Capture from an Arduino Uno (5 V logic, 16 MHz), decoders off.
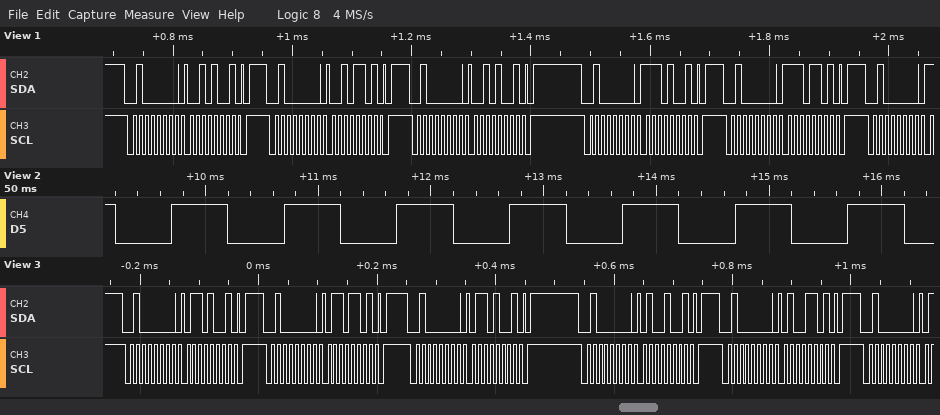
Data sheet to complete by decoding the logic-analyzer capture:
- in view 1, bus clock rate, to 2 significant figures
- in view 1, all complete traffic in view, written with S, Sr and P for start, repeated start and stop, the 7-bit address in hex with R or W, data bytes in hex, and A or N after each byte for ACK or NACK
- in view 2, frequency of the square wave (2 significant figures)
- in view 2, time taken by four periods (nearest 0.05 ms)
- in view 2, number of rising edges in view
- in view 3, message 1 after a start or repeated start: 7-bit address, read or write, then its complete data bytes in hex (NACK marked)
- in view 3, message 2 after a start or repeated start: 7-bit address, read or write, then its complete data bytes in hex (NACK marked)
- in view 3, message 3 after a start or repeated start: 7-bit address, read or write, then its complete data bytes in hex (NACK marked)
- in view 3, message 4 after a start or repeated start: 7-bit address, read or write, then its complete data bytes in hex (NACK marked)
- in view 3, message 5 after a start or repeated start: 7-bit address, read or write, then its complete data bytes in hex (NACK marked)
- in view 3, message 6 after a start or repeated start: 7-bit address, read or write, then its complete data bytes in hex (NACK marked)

100 kHz
S 20W A 29 A P S 20W A 2D A P S 20W A 29 A P S 20W A E9 A P S 20W A ED A P S 20W A
1.0 kHz
4.00 ms
7
0x20 write: 69
0x20 write: 6D
0x20 write: 69
0x20 write: 49
0x20 write: 4D
0x20 write
